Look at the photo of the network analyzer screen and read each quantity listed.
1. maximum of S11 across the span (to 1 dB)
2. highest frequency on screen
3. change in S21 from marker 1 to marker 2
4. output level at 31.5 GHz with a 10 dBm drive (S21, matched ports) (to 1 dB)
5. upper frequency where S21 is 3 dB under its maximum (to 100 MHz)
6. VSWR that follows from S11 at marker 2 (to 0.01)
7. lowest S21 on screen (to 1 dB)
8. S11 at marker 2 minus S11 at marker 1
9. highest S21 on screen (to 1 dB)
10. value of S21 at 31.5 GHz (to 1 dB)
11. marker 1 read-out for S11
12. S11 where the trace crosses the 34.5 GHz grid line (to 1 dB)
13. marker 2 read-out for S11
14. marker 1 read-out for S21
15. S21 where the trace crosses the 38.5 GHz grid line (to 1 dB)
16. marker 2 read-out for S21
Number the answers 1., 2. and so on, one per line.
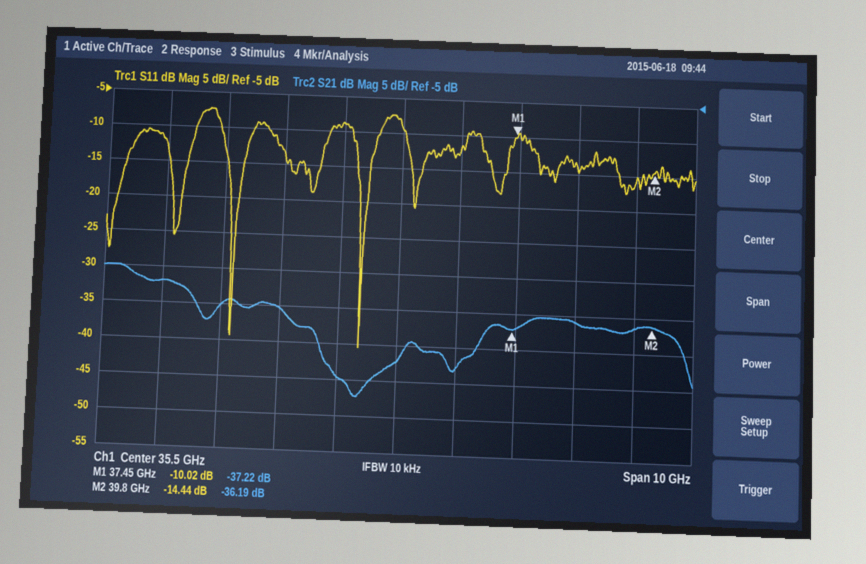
1. -7 dB
2. 40.5 GHz
3. 1.03 dB
4. -22 dBm
5. 31.9 GHz
6. 1.47
7. -47 dB
8. -4.42 dB
9. -30 dB
10. -32 dB
11. -10.02 dB
12. -9 dB
13. -14.44 dB
14. -37.22 dB
15. -36 dB
16. -36.19 dB
